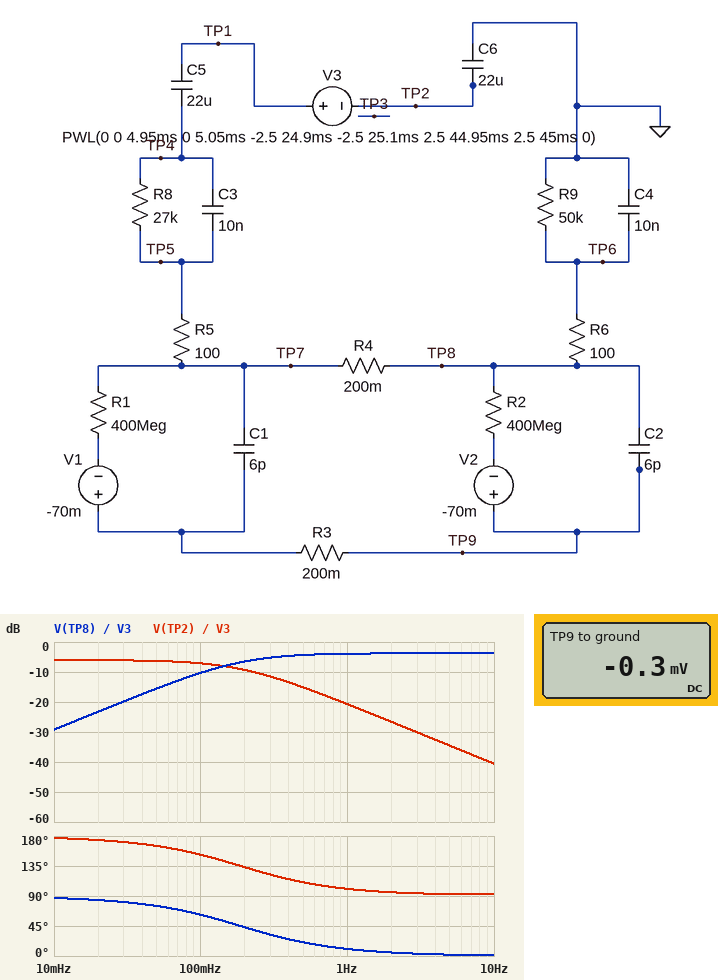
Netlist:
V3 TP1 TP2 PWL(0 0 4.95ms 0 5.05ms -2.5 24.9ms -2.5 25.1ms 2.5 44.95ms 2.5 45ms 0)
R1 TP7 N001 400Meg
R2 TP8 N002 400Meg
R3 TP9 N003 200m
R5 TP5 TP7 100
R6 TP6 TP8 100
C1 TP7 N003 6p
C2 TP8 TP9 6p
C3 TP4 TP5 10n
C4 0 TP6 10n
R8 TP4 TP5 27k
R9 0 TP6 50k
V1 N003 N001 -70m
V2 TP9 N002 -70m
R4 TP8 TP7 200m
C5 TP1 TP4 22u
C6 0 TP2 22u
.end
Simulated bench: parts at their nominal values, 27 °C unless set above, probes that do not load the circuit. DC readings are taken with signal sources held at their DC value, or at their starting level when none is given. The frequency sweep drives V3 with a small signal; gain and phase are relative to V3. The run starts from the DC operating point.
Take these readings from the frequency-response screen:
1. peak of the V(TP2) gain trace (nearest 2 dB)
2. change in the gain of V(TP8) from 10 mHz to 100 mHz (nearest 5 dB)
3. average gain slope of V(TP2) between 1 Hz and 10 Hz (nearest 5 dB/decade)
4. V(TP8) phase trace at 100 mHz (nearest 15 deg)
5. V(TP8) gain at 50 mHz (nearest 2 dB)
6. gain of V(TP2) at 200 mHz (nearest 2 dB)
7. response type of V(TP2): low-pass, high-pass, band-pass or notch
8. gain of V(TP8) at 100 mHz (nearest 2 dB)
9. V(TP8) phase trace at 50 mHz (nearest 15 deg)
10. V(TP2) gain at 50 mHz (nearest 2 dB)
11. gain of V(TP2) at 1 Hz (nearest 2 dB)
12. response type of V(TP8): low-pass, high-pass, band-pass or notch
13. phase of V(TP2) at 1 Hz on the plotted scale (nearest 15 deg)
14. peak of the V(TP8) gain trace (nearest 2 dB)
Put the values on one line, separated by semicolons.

-6 dB; 20 dB; -20 dB/decade; 60 deg; -16 dB; -10 dB; low-pass; -10 dB; 75 deg; -6 dB; -20 dB; high-pass; 105 deg; -4 dB
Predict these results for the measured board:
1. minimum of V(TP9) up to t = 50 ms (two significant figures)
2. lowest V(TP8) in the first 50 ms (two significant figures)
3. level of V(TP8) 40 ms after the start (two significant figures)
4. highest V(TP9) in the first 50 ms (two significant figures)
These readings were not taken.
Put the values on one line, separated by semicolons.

-1.7 V; -1.6 V; 1.6 V; 1.6 V
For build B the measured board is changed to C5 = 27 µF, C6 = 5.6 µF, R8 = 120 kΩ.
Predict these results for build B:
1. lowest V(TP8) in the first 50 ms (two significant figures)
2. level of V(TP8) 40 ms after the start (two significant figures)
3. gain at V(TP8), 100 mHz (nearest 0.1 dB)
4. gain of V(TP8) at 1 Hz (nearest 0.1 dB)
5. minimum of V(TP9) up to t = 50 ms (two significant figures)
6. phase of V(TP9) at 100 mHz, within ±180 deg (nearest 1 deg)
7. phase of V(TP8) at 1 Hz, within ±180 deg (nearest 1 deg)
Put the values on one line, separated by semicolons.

-1.2 V; 740 mV; -17.7 dB; -10.8 dB; -1.3 V; 64 deg; 12 deg
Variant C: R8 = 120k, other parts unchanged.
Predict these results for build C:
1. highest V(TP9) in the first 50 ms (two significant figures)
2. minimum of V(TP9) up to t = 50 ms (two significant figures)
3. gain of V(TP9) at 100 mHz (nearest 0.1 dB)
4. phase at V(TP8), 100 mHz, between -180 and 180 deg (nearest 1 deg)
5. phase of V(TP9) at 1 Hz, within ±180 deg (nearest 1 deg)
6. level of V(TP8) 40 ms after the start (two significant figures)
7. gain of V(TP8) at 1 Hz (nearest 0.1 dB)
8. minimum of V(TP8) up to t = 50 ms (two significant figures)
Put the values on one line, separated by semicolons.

1.6 V; -1.3 V; -13.0 dB; 40 deg; 5 deg; 740 mV; -10.7 dB; -1.2 V
